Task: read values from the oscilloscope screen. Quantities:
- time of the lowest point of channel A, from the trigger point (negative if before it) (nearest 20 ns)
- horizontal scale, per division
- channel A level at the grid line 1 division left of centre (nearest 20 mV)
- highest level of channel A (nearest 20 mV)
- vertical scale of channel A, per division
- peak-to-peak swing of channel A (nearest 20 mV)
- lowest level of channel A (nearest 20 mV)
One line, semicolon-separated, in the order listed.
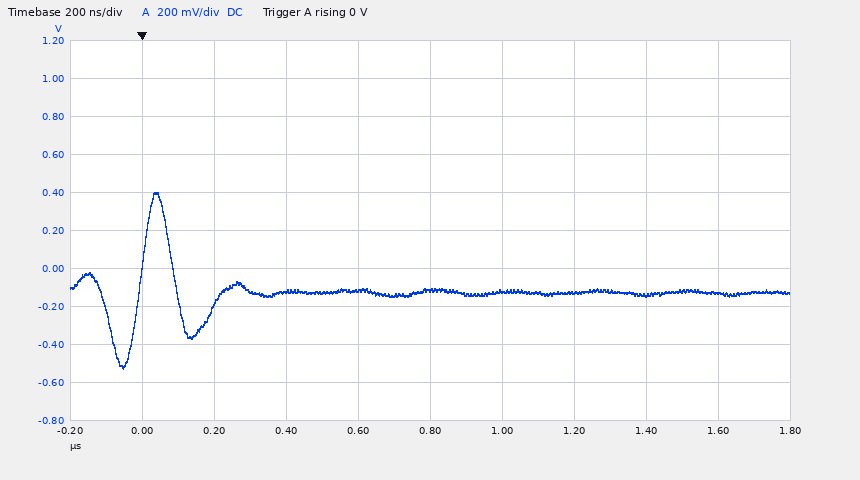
-60 ns; 200 ns; -120 mV; 400 mV; 200 mV; 920 mV; -520 mV
